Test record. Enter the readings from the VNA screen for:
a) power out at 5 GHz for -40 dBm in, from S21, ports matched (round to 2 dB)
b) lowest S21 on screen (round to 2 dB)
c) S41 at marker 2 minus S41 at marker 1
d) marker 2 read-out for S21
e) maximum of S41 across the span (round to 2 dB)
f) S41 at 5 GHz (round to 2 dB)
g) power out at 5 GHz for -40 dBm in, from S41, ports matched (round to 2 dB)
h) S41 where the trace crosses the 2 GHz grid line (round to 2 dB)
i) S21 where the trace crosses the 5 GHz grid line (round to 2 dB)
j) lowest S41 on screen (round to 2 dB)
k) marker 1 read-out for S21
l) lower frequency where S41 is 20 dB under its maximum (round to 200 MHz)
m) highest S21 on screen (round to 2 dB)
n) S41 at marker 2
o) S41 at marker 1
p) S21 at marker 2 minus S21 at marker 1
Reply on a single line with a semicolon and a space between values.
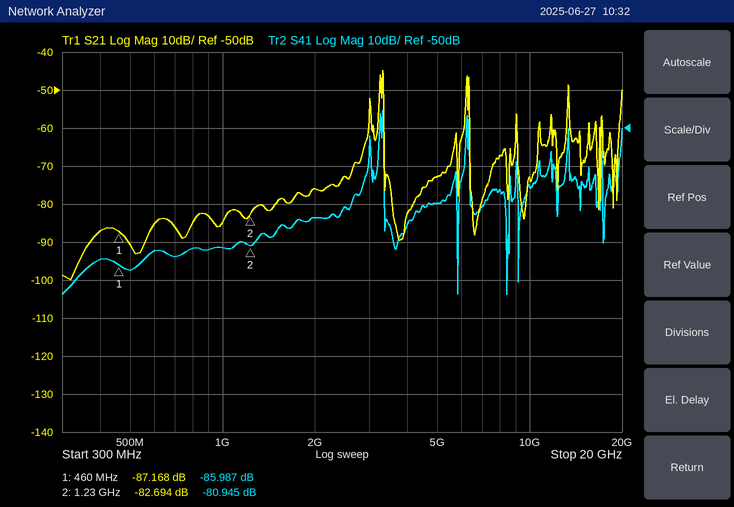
-112 dBm; -100 dB; 5.042 dB; -82.694 dB; -46 dB; -70 dB; -110 dBm; -74 dB; -72 dB; -94 dB; -87.168 dB; 2.8 GHz; -44 dB; -80.945 dB; -85.987 dB; 4.474 dB
